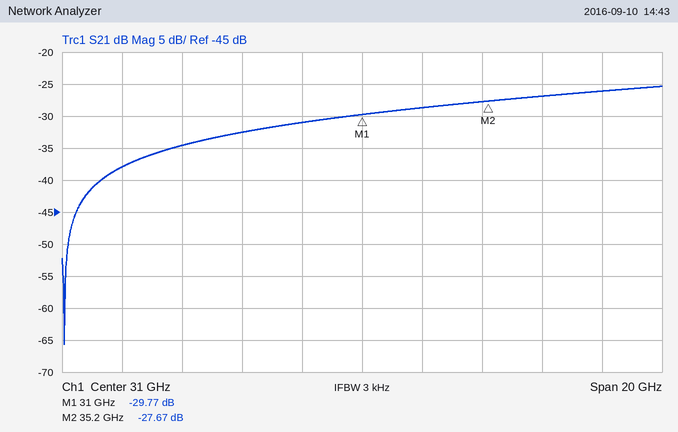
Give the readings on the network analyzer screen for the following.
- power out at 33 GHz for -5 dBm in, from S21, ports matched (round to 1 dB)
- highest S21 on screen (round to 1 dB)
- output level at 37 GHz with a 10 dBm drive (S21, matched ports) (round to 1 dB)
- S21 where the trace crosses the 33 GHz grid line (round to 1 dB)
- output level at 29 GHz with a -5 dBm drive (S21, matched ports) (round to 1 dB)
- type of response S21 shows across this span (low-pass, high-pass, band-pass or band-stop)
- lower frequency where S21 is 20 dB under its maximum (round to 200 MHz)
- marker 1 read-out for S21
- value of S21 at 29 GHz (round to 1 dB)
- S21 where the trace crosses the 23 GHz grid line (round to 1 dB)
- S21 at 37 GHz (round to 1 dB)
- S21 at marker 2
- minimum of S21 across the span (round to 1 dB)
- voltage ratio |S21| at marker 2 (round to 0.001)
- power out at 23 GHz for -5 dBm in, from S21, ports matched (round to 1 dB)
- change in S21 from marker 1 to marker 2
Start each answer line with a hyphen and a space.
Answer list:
- -34 dBm
- -25 dB
- -17 dBm
- -29 dB
- -36 dBm
- high-pass
- 21.4 GHz
- -29.77 dB
- -31 dB
- -38 dB
- -27 dB
- -27.67 dB
- -66 dB
- 0.041
- -43 dBm
- 2.10 dB
